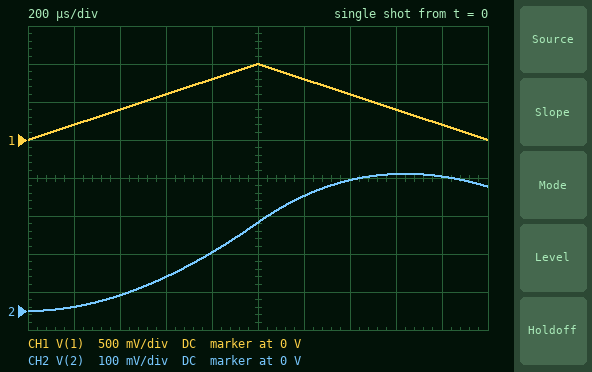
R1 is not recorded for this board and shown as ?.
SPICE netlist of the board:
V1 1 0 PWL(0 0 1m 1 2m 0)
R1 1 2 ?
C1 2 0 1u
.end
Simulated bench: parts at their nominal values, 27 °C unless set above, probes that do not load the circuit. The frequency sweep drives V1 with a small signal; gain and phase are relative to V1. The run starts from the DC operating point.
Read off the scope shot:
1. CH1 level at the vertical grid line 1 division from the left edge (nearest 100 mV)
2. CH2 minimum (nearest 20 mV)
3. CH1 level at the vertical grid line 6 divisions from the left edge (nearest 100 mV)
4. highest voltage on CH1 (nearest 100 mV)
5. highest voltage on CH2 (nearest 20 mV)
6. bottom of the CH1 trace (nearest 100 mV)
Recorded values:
200 mV
0 V
800 mV
1.0 V
360 mV
0 V
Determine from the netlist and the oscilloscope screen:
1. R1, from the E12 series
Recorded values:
1.8 kΩ
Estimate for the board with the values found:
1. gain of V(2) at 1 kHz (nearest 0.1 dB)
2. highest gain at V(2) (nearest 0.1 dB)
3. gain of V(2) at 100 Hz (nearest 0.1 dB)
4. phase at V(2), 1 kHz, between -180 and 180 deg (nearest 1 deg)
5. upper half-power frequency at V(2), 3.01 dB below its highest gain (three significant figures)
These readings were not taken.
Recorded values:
-21.1 dB
0 dB
-3.6 dB
-85 deg
88.4 Hz
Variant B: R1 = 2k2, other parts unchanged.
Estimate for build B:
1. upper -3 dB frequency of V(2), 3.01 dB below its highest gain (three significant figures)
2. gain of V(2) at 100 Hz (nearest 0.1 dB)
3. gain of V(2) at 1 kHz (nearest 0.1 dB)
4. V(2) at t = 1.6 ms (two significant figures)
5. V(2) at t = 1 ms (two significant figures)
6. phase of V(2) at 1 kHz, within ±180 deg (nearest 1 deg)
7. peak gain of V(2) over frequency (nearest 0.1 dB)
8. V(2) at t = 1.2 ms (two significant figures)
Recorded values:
72.3 Hz
-4.6 dB
-22.8 dB
310 mV
200 mV
-86 deg
0 dB
260 mV
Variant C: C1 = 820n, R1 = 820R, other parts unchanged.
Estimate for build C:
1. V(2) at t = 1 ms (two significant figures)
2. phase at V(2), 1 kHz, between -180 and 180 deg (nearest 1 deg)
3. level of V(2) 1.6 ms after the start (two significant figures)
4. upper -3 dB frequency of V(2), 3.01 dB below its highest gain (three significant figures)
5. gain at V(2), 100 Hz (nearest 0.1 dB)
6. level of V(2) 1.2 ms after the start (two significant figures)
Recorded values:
480 mV
-77 deg
580 mV
237 Hz
-0.7 dB
590 mV
